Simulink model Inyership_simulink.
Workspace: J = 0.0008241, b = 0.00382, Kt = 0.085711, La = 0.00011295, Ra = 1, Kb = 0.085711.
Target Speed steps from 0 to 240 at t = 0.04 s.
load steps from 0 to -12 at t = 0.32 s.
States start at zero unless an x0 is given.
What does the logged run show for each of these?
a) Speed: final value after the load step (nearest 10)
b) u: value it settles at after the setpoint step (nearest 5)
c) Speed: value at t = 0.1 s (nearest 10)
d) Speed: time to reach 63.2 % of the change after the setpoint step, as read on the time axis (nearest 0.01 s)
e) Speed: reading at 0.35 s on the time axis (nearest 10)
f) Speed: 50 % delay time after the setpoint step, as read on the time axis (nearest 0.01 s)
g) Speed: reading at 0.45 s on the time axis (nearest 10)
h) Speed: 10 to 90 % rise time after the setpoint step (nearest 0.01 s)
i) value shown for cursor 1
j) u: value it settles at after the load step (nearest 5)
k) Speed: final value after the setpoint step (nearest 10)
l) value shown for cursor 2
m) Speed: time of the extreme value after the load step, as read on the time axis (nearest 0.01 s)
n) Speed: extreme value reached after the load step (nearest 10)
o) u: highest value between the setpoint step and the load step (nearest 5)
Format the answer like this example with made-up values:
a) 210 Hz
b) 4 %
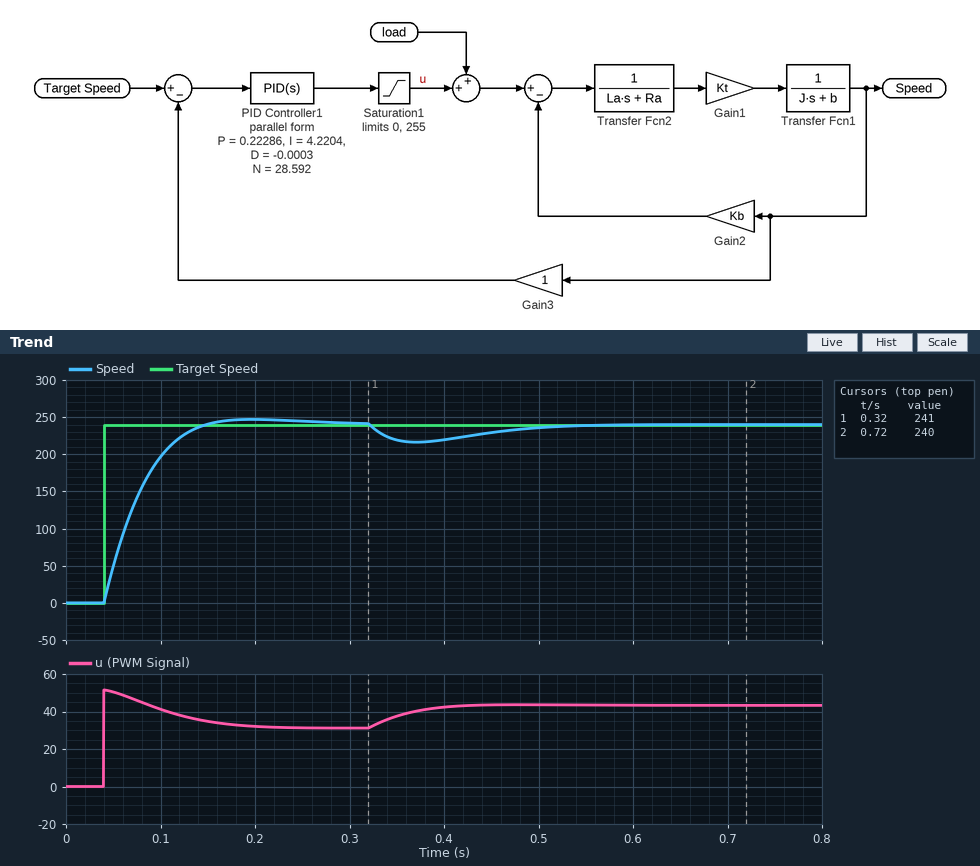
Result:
a) 240
b) 30
c) 200
d) 0.08 s
e) 220
f) 0.07 s
g) 230
h) 0.07 s
i) 241
j) 45
k) 240
l) 240
m) 0.37 s
n) 220
o) 50
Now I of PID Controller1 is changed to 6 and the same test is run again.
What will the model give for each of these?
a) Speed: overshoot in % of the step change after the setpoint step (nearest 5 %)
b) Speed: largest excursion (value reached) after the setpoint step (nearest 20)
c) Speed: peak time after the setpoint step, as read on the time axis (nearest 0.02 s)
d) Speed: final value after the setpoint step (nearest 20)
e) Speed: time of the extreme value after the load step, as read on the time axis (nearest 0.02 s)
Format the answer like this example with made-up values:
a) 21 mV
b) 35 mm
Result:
a) 10 %
b) 260
c) 0.16 s
d) 240
e) 0.36 s
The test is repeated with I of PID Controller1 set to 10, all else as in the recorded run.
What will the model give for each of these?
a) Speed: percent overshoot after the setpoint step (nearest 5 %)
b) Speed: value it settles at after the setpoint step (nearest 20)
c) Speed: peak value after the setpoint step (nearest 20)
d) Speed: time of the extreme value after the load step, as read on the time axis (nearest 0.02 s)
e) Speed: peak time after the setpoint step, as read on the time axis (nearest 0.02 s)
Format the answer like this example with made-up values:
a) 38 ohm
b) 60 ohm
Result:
a) 15 %
b) 240
c) 280
d) 0.36 s
e) 0.12 s
